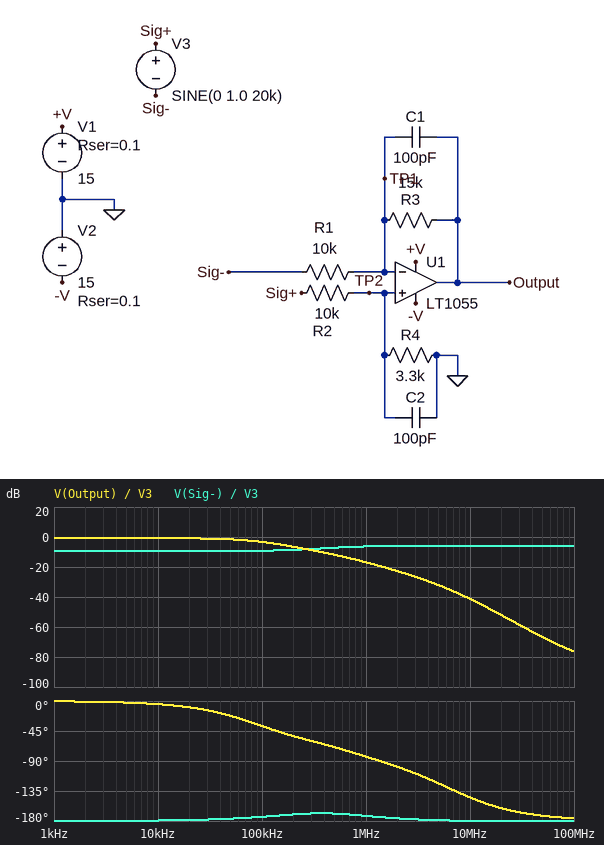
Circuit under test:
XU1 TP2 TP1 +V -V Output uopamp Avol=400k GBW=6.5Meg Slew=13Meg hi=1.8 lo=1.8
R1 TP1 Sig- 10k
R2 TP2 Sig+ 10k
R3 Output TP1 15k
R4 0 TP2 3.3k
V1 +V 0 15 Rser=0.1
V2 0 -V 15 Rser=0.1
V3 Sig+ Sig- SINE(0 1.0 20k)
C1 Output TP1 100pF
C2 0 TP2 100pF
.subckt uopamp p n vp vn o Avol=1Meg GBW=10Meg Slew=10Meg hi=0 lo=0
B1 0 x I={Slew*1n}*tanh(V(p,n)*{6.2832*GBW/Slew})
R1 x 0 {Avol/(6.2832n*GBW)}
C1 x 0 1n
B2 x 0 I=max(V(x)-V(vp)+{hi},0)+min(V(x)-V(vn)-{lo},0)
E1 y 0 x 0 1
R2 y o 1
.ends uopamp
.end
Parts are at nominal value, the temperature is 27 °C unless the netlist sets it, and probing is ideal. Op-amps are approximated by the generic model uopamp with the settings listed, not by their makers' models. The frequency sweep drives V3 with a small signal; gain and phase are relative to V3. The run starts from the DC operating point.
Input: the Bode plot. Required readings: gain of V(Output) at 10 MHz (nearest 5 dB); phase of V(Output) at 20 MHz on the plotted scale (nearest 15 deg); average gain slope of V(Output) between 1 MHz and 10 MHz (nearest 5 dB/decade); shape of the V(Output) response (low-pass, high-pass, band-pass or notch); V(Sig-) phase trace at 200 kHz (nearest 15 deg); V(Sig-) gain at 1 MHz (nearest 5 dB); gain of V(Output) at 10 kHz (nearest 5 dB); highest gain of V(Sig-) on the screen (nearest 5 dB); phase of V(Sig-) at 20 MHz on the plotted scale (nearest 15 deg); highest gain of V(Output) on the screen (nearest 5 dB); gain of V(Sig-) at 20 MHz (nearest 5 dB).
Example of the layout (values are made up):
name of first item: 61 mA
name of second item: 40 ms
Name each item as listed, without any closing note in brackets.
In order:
gain of V(Output) at 10 MHz: -40 dB
phase of V(Output) at 20 MHz on the plotted scale: -165 deg
average gain slope of V(Output) between 1 MHz and 10 MHz: -25 dB/decade
shape of the V(Output) response: low-pass
V(Sig-) phase trace at 200 kHz: -165 deg
V(Sig-) gain at 1 MHz: -5 dB
gain of V(Output) at 10 kHz: 0 dB
highest gain of V(Sig-) on the screen: -5 dB
phase of V(Sig-) at 20 MHz on the plotted scale: -180 deg
highest gain of V(Output) on the screen: 0 dB
gain of V(Sig-) at 20 MHz: -5 dB
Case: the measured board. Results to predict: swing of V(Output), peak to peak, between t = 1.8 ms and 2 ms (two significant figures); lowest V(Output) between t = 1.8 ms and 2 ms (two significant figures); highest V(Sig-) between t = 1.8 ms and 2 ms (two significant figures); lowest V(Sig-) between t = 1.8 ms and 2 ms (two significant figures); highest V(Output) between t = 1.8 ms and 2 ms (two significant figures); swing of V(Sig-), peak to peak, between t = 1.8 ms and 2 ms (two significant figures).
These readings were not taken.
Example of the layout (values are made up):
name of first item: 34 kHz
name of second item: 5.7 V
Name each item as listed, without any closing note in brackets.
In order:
swing of V(Output), peak to peak, between t = 1.8 ms and 2 ms: 1.8 V
lowest V(Output) between t = 1.8 ms and 2 ms: -900 mV
highest V(Sig-) between t = 1.8 ms and 2 ms: 340 mV
lowest V(Sig-) between t = 1.8 ms and 2 ms: -340 mV
highest V(Output) between t = 1.8 ms and 2 ms: 900 mV
swing of V(Sig-), peak to peak, between t = 1.8 ms and 2 ms: 670 mV
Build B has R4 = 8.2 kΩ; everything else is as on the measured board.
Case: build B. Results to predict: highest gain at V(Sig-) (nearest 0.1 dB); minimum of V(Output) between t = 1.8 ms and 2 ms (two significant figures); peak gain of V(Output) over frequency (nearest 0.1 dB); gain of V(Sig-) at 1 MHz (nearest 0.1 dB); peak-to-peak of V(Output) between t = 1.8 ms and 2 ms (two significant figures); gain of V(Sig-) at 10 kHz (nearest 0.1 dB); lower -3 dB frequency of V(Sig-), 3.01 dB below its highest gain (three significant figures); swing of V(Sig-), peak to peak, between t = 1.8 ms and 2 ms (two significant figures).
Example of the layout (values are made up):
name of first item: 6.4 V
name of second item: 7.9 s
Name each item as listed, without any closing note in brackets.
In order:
highest gain at V(Sig-): -5.9 dB
minimum of V(Output) between t = 1.8 ms and 2 ms: -1.1 V
peak gain of V(Output) over frequency: 1.3 dB
gain of V(Sig-) at 1 MHz: -6.0 dB
peak-to-peak of V(Output) between t = 1.8 ms and 2 ms: 2.3 V
gain of V(Sig-) at 10 kHz: -20.5 dB
lower -3 dB frequency of V(Sig-), 3.01 dB below its highest gain: 180 kHz
swing of V(Sig-), peak to peak, between t = 1.8 ms and 2 ms: 210 mV
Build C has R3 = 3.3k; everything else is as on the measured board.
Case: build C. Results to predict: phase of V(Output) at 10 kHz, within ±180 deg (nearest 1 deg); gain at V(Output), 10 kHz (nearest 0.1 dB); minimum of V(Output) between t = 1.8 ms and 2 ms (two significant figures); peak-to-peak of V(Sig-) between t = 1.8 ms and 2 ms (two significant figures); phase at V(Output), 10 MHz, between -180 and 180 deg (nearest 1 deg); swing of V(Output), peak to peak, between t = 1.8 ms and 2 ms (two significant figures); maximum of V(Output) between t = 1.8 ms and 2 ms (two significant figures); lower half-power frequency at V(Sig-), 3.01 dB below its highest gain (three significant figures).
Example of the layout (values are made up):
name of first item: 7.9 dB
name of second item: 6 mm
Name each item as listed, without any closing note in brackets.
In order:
phase of V(Output) at 10 kHz, within ±180 deg: -1 deg
gain at V(Output), 10 kHz: -9.6 dB
minimum of V(Output) between t = 1.8 ms and 2 ms: -330 mV
peak-to-peak of V(Sig-) between t = 1.8 ms and 2 ms: 670 mV
phase at V(Output), 10 MHz, between -180 and 180 deg: -144 deg
swing of V(Output), peak to peak, between t = 1.8 ms and 2 ms: 660 mV
maximum of V(Output) between t = 1.8 ms and 2 ms: 330 mV
lower half-power frequency at V(Sig-), 3.01 dB below its highest gain: 164 kHz
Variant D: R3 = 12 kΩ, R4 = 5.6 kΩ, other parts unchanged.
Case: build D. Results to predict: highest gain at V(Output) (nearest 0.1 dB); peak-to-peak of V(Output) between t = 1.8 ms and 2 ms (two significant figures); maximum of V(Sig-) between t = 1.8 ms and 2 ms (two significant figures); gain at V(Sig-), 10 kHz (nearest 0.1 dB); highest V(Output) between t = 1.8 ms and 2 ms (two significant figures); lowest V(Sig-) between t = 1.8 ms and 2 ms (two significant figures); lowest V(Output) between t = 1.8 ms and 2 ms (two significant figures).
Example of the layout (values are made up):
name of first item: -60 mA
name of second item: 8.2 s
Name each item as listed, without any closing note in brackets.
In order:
highest gain at V(Output): -1.1 dB
peak-to-peak of V(Output) between t = 1.8 ms and 2 ms: 1.7 V
maximum of V(Sig-) between t = 1.8 ms and 2 ms: 220 mV
gain at V(Sig-), 10 kHz: -13.1 dB
highest V(Output) between t = 1.8 ms and 2 ms: 870 mV
lowest V(Sig-) between t = 1.8 ms and 2 ms: -220 mV
lowest V(Output) between t = 1.8 ms and 2 ms: -870 mV
